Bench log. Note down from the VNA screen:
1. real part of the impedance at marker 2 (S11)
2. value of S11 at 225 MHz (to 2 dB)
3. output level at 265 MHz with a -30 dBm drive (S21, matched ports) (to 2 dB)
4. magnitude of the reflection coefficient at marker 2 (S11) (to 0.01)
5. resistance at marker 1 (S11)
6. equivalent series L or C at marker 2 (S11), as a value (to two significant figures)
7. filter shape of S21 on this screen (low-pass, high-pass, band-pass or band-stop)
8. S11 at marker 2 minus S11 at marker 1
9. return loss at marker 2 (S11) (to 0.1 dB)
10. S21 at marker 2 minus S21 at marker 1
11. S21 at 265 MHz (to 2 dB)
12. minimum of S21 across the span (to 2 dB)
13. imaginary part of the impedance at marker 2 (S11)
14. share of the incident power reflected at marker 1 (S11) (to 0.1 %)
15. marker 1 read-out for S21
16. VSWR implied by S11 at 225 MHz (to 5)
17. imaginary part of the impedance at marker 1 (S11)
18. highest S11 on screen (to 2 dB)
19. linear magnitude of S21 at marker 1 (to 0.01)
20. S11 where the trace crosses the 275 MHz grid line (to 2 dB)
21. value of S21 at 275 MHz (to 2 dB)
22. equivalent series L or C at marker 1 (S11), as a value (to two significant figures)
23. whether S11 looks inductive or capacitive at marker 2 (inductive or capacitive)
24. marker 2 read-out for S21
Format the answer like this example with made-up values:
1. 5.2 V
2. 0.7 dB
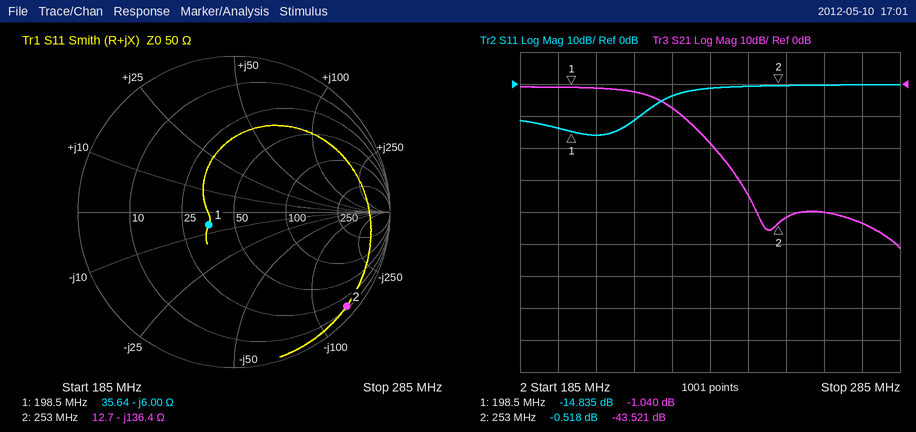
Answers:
1. 12.7 Ω
2. -4 dB
3. -70 dBm
4. 0.94
5. 35.64 Ω
6. 4.6 pF
7. low-pass
8. 14.317 dB
9. 0.5 dB
10. -42.481 dB
11. -40 dB
12. -52 dB
13. -136.4 Ω
14. 3.3 %
15. -1.040 dB
16. 5
17. -6.00 Ω
18. 0 dB
19. 0.89
20. 0 dB
21. -44 dB
22. 130 pF
23. capacitive
24. -43.521 dB
